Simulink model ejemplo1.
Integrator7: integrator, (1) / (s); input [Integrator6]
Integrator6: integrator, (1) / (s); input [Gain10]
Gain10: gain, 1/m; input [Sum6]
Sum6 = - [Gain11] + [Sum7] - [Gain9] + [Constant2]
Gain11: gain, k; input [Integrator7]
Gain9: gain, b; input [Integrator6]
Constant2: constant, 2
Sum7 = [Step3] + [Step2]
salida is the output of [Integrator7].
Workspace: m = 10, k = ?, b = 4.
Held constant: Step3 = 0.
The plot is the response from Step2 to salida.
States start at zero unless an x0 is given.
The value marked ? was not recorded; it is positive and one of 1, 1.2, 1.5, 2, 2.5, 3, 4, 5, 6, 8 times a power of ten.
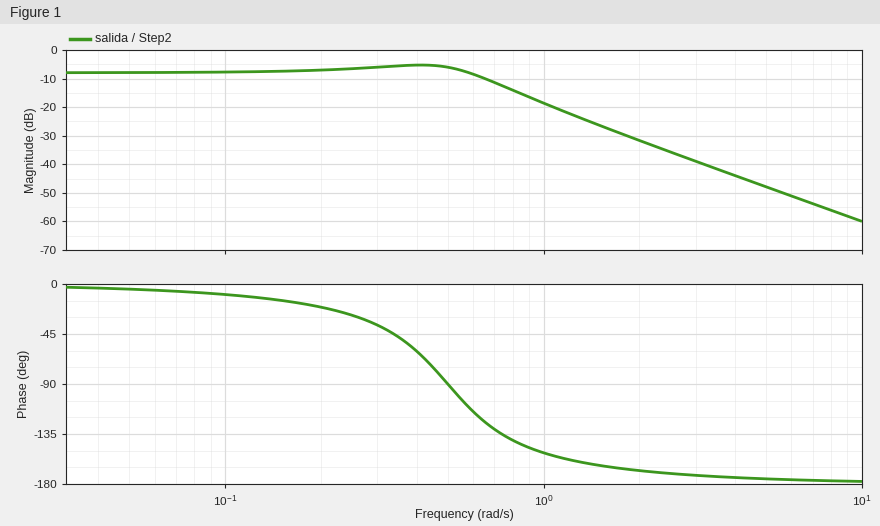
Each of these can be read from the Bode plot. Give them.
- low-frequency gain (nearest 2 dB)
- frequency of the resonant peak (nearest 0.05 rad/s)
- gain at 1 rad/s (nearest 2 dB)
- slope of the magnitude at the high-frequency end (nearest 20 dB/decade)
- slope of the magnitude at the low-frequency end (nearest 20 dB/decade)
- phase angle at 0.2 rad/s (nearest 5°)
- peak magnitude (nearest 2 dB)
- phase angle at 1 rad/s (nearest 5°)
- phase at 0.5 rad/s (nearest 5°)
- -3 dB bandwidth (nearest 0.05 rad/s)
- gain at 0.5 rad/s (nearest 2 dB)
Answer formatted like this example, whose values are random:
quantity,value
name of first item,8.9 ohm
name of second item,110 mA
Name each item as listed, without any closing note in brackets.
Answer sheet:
quantity,value
low-frequency gain,-8 dB
frequency of the resonant peak,0.40 rad/s
gain at 1 rad/s,-18 dB
slope of the magnitude at the high-frequency end,-40 dB/decade
slope of the magnitude at the low-frequency end,0 dB/decade
phase angle at 0.2 rad/s,-20°
peak magnitude,-6 dB
phase angle at 1 rad/s,-150°
phase at 0.5 rad/s,-90°
-3 dB bandwidth,0.70 rad/s
gain at 0.5 rad/s,-6 dB
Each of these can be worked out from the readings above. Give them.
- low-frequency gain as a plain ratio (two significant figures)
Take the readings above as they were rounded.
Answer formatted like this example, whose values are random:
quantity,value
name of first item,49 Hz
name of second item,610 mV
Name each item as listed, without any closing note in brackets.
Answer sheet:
quantity,value
low-frequency gain as a plain ratio,0.40
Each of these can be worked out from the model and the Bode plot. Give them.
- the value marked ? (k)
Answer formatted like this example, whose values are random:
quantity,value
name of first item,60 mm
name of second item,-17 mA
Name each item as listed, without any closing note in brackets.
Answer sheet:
quantity,value
the value marked ?,2.5
